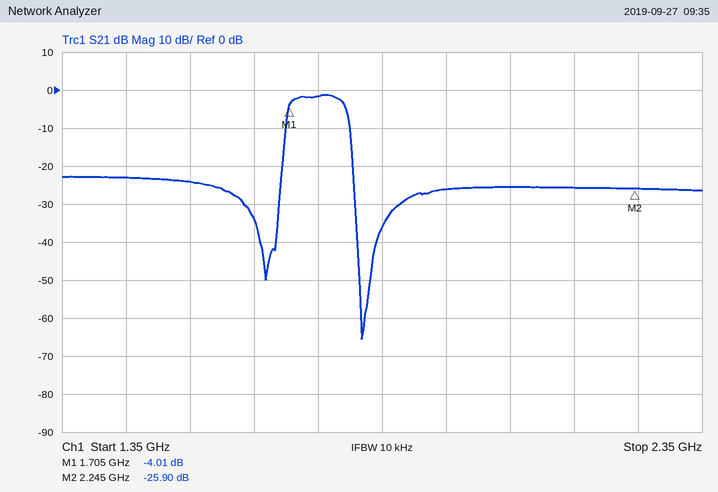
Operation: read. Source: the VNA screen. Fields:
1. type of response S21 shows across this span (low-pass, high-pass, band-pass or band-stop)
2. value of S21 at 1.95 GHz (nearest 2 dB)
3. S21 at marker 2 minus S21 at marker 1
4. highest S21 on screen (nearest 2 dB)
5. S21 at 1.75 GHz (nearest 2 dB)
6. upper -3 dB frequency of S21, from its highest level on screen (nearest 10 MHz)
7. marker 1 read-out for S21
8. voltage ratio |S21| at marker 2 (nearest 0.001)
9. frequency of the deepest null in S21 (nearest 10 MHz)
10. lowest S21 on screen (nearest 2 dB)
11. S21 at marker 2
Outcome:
band-pass
-26 dB
-21.89 dB
-2 dB
-2 dB
1.79 GHz
-4.01 dB
0.051
1.82 GHz
-66 dB
-25.90 dB
